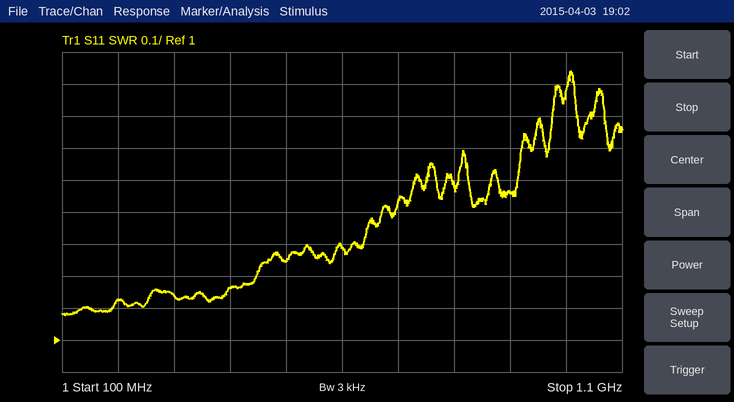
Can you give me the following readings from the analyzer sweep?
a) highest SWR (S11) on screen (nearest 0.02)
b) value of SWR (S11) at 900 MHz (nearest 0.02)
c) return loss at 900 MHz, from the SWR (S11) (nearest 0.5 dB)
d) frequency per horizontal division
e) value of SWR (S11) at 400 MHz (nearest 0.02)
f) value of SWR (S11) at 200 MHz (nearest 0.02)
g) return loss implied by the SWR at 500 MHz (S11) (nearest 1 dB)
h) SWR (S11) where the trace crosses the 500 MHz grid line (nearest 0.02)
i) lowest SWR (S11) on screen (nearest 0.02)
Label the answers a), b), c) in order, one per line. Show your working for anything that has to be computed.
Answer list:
a) 1.84
b) 1.46
c) −20 log10((1.46 − 1)/(1.46 + 1)) ≈ 14.6 dB, so 14.5 dB to the nearest 0.5 dB
d) 100 MHz
e) 1.16
f) 1.12
g) −20 log10((1.24 − 1)/(1.24 + 1)) ≈ 19 dB
h) 1.24
i) 1.08
